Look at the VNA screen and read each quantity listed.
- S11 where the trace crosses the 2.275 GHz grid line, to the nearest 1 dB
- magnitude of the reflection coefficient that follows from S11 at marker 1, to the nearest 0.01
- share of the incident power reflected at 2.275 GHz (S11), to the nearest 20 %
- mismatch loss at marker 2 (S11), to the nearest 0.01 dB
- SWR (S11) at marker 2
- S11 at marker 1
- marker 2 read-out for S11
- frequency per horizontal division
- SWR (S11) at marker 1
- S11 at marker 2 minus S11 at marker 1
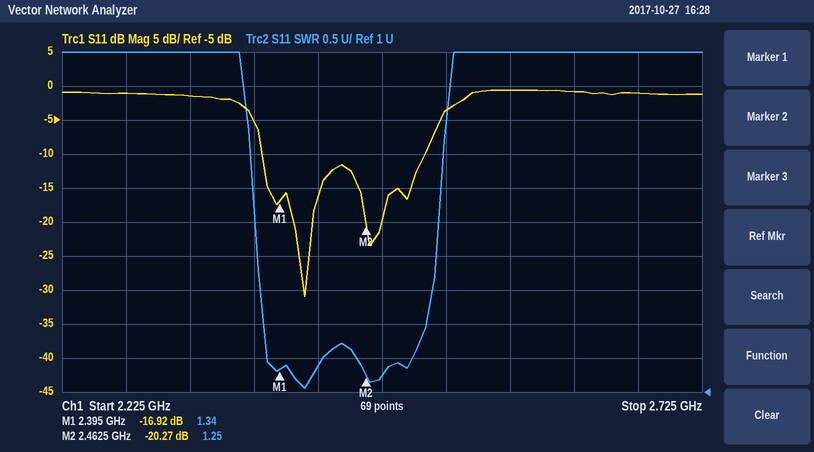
-1 dB
0.14
80 %
0.04 dB
1.25
-16.92 dB
-20.27 dB
50 MHz
1.34
-3.35 dB
